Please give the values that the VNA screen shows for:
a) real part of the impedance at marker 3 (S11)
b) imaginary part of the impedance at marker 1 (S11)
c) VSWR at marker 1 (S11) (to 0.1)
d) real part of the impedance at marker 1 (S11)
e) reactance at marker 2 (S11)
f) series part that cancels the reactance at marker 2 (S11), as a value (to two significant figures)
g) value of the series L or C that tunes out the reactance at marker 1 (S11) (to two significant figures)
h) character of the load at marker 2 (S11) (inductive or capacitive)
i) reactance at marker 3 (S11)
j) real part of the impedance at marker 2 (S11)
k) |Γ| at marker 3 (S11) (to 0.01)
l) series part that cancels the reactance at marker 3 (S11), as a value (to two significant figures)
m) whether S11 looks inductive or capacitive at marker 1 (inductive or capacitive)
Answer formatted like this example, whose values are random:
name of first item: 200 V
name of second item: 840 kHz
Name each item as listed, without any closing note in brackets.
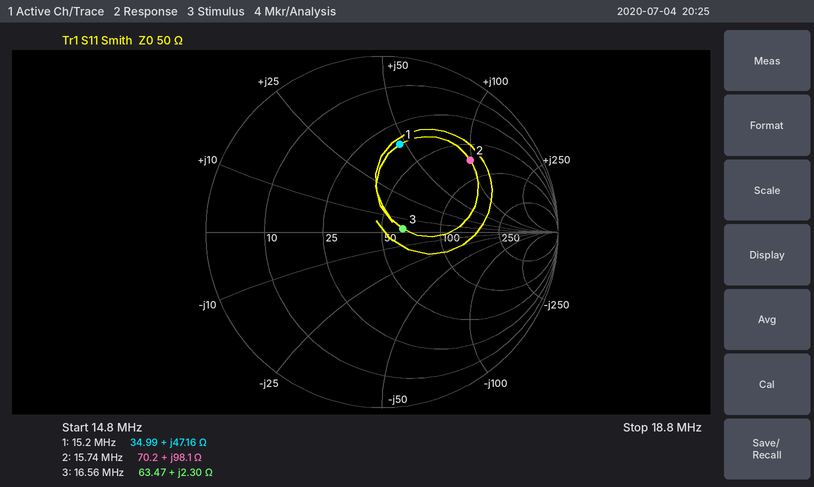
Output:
real part of the impedance at marker 3: 63.47 Ω
imaginary part of the impedance at marker 1: +47.16 Ω
VSWR at marker 1 (S11): 3.1
real part of the impedance at marker 1: 34.99 Ω
reactance at marker 2: +98.1 Ω
series part that cancels the reactance at marker 2 (S11), as a value: 100 pF
value of the series L or C that tunes out the reactance at marker 1 (S11): 220 pF
character of the load at marker 2 (S11): inductive
reactance at marker 3: +2.30 Ω
real part of the impedance at marker 2: 70.2 Ω
|Γ| at marker 3 (S11): 0.12
series part that cancels the reactance at marker 3 (S11), as a value: 4.2 nF
whether S11 looks inductive or capacitive at marker 1: inductive
